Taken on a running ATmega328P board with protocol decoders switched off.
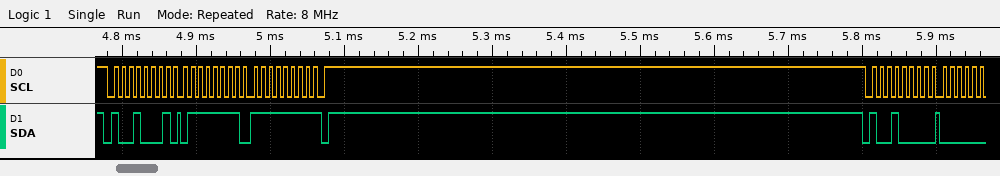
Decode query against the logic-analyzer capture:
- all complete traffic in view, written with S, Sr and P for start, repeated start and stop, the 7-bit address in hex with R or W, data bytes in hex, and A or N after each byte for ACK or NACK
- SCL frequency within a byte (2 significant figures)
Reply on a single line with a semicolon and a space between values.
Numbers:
S 48R A 7F A FF N P S 48W A; 100 kHz
